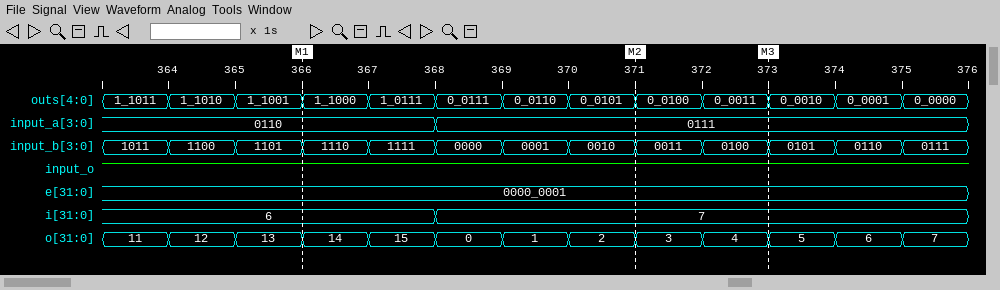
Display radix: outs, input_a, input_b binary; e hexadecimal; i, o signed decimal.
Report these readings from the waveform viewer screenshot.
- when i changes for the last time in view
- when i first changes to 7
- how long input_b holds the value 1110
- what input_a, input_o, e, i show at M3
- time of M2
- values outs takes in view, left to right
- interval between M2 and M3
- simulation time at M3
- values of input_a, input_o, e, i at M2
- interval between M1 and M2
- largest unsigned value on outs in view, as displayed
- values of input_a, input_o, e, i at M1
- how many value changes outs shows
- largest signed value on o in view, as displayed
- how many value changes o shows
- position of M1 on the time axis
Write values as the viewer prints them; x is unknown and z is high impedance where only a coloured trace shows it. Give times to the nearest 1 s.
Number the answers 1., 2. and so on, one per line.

1. 368 s
2. 368 s
3. 1 s
4. input_a=0111, input_o=1, e=0000_0001, i=7
5. 371 s
6. 1_1011, 1_1010, 1_1001, 1_1000, 1_0111, 0_0111, 0_0110, 0_0101, 0_0100, 0_0011, 0_0010, 0_0001, 0_0000
7. 2 s
8. 373 s
9. input_a=0111, input_o=1, e=0000_0001, i=7
10. 5 s
11. 1_1011
12. input_a=0110, input_o=1, e=0000_0001, i=6
13. 12
14. 15
15. 12
16. 366 s
